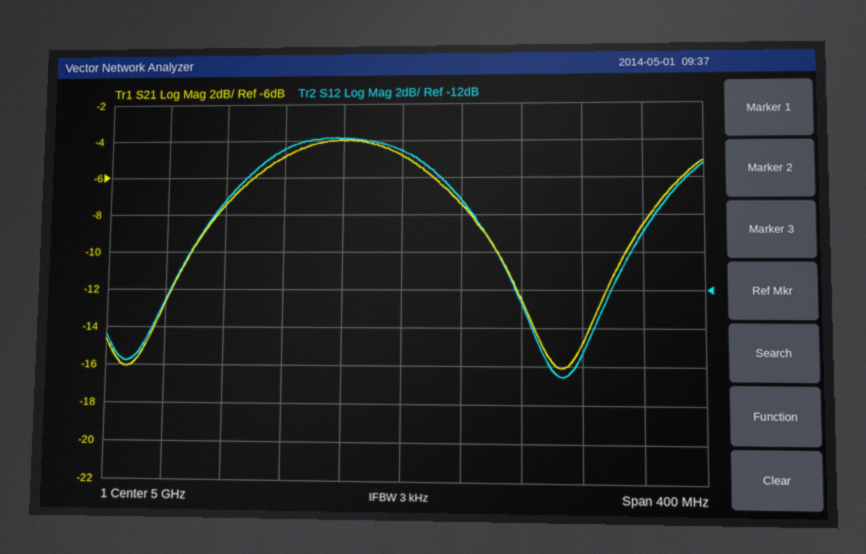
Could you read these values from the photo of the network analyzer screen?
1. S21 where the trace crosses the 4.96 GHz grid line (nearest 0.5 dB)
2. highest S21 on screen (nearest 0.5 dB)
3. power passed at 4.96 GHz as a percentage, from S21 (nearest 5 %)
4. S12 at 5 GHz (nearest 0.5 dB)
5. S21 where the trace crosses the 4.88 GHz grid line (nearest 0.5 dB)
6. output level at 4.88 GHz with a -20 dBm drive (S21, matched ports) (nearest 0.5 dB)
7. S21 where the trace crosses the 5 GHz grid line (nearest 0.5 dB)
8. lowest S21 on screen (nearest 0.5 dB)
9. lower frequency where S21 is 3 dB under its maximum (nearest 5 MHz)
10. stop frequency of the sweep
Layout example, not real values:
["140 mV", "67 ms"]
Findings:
["-4.0 dB", "-4.0 dB", "40 %", "-4.5 dB", "-7.5 dB", "-27.5 dBm", "-5.0 dB", "-16.0 dB", "4.885 GHz", "5.2 GHz"]
